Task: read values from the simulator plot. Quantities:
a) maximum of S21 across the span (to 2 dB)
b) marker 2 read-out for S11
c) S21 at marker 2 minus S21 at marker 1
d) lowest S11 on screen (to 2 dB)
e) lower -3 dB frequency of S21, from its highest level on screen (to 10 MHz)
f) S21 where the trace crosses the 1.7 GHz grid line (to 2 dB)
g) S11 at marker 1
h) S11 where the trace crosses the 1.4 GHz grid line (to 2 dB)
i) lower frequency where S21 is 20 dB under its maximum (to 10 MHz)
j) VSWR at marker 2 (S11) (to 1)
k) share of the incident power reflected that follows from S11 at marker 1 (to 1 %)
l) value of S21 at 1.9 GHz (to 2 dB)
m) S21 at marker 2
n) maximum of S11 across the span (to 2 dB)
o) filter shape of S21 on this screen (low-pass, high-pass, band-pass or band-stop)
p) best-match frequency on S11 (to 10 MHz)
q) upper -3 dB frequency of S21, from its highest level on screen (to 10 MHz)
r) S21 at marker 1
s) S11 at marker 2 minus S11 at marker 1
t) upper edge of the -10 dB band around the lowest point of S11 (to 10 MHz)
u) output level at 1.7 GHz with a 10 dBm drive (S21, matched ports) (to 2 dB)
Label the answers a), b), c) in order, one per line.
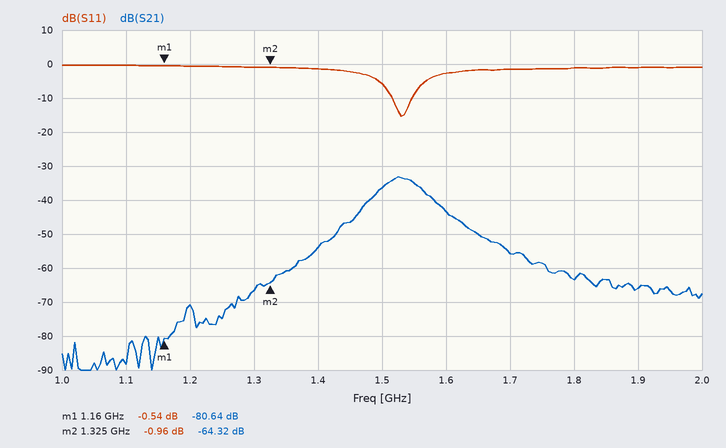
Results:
a) -34 dB
b) -0.96 dB
c) 16.32 dB
d) -16 dB
e) 1.50 GHz
f) -56 dB
g) -0.54 dB
h) -2 dB
i) 1.40 GHz
j) 18
k) 88 %
l) -66 dB
m) -64.32 dB
n) 0 dB
o) band-pass
p) 1.53 GHz
q) 1.56 GHz
r) -80.64 dB
s) -0.42 dB
t) 1.55 GHz
u) -46 dBm
